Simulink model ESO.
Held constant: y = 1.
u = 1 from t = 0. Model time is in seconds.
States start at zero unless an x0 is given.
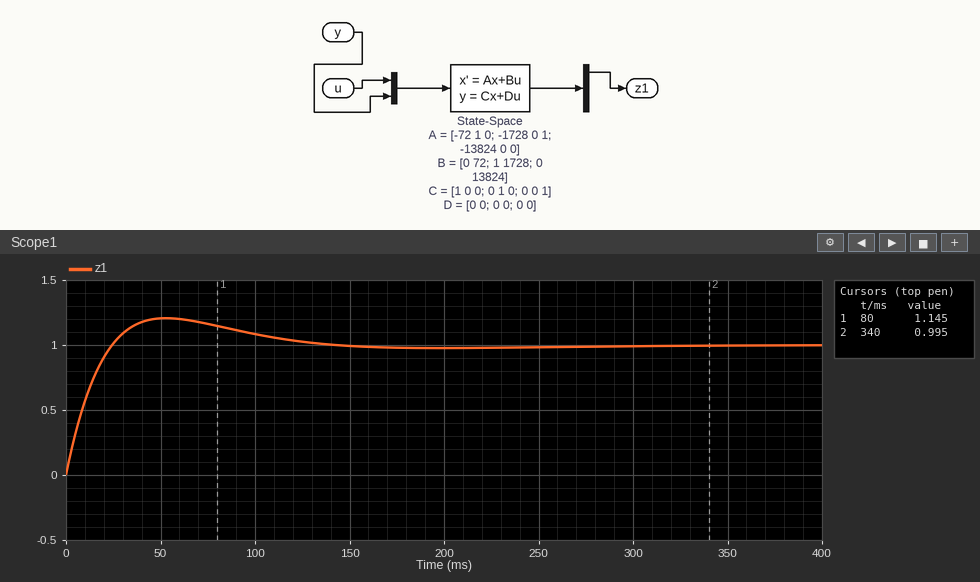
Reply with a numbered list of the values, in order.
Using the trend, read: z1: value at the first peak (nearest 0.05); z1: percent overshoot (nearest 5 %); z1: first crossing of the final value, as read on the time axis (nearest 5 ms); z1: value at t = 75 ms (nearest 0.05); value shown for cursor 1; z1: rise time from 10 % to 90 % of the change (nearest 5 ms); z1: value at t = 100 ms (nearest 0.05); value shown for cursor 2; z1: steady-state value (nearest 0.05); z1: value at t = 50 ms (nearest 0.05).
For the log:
1. 1.20
2. 20 %
3. 25 ms
4. 1.15
5. 1.145
6. 20 ms
7. 1.10
8. 0.995
9. 1.00
10. 1.20
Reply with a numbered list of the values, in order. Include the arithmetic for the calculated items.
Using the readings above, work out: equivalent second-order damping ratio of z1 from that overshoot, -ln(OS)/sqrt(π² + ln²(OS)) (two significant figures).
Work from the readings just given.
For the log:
1. ln(0.2) = -1.609; 1.609 / sqrt(9.870 + 2.590) = 0.46
